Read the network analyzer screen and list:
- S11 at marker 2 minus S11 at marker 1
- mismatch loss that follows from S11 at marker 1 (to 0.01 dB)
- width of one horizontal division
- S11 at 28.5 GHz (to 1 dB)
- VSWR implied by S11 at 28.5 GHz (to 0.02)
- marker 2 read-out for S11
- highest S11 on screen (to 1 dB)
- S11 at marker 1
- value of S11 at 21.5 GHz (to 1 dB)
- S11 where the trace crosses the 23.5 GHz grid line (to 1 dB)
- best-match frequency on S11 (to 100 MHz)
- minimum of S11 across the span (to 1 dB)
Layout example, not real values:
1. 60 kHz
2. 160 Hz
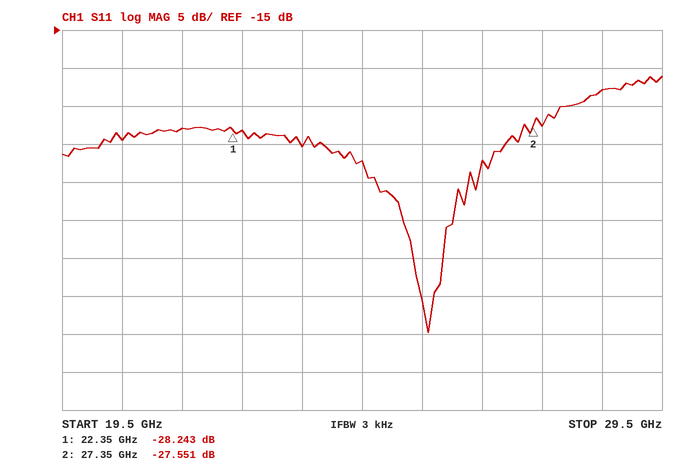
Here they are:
1. 0.692 dB
2. 0.01 dB
3. 1 GHz
4. -23 dB
5. 1.16
6. -27.551 dB
7. -21 dB
8. -28.243 dB
9. -28 dB
10. -30 dB
11. 25.6 GHz
12. -55 dB
